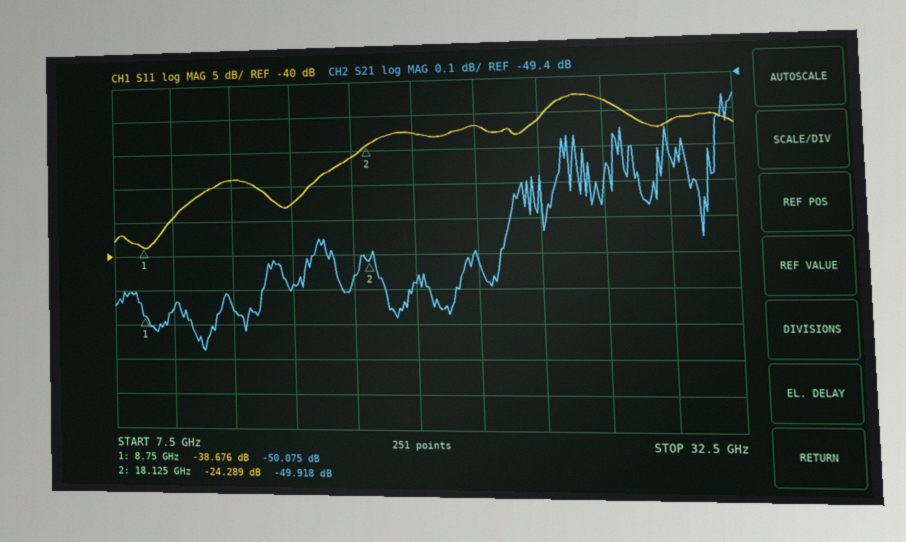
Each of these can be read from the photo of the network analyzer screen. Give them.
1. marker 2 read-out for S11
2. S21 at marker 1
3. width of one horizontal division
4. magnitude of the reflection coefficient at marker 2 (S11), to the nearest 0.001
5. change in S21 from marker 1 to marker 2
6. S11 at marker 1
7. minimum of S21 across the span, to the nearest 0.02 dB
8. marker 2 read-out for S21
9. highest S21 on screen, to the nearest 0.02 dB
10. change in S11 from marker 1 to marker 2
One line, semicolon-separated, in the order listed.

-24.289 dB; -50.075 dB; 2.5 GHz; 0.061; 0.157 dB; -38.676 dB; -50.18 dB; -49.918 dB; -49.46 dB; 14.387 dB
